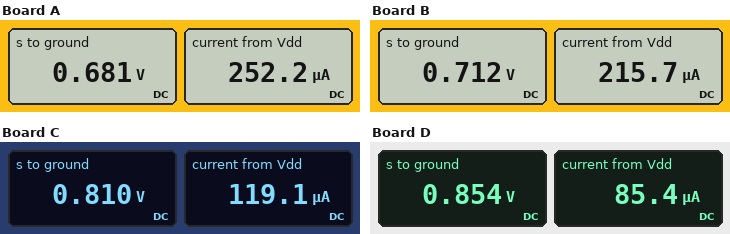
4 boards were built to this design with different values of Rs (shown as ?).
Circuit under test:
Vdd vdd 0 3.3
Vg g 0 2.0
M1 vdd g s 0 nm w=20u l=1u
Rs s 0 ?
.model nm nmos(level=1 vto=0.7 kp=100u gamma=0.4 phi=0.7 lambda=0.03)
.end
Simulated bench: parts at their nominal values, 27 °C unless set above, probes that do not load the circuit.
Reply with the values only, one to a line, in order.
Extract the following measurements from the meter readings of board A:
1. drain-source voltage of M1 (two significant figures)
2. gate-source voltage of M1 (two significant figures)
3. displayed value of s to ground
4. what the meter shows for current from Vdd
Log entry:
2.6 V
1.3 V
0.681 V
252.2 µA
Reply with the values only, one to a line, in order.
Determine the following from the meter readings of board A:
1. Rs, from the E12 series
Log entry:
2.7 kΩ
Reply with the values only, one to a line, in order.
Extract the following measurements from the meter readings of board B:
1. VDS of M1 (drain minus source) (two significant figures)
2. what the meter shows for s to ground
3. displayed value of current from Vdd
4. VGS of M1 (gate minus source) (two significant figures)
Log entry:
2.6 V
0.712 V
215.7 µA
1.3 V
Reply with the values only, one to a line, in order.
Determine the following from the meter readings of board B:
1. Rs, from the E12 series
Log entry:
3.3 kΩ
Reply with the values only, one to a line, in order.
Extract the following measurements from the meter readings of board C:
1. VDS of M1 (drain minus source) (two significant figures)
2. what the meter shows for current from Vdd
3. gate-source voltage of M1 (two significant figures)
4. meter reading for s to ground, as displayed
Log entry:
2.5 V
119.1 µA
1.2 V
0.810 V
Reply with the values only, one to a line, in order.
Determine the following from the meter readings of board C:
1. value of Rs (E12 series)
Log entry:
6.8 kΩ
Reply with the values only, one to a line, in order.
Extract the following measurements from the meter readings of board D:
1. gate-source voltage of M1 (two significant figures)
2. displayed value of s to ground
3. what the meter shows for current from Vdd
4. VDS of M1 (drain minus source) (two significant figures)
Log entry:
1.1 V
0.854 V
85.4 µA
2.4 V
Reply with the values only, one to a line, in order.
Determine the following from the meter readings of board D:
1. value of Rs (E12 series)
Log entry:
10 kΩ
